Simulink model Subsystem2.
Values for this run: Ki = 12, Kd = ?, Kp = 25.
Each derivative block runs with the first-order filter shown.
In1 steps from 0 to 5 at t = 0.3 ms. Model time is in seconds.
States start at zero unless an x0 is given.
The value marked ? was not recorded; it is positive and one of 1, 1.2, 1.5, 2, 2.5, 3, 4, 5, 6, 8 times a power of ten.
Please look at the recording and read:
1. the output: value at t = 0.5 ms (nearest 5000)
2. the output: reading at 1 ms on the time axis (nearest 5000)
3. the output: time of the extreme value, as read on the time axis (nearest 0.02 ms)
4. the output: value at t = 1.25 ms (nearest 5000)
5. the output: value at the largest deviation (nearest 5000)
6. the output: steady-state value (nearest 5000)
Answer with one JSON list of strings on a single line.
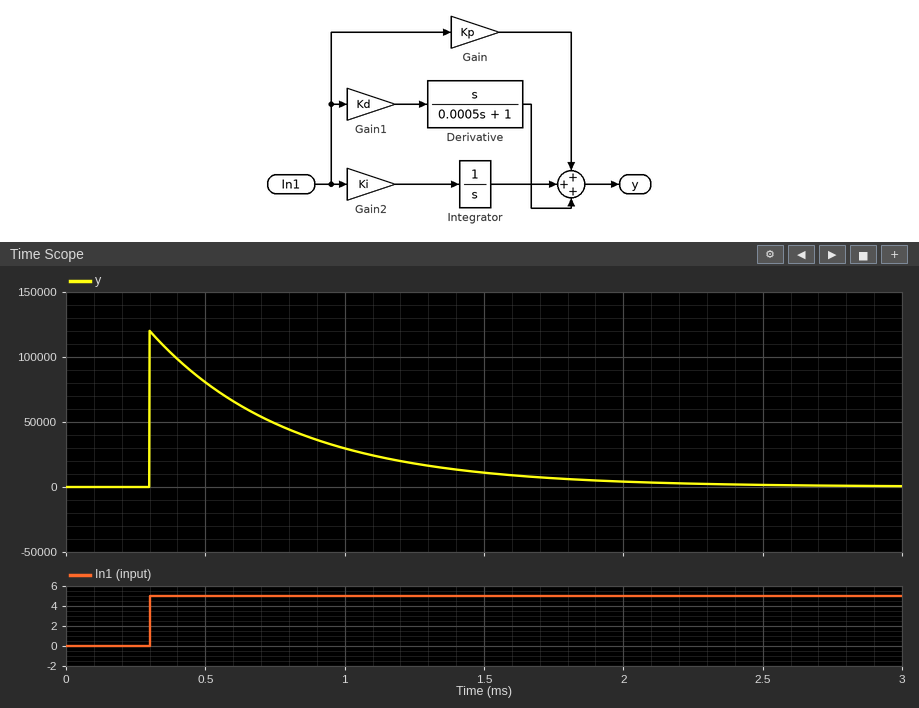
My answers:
["80000", "30000", "0.30 ms", "20000", "120000", "0"]
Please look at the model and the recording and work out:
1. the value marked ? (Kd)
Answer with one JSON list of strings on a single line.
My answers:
["12"]
